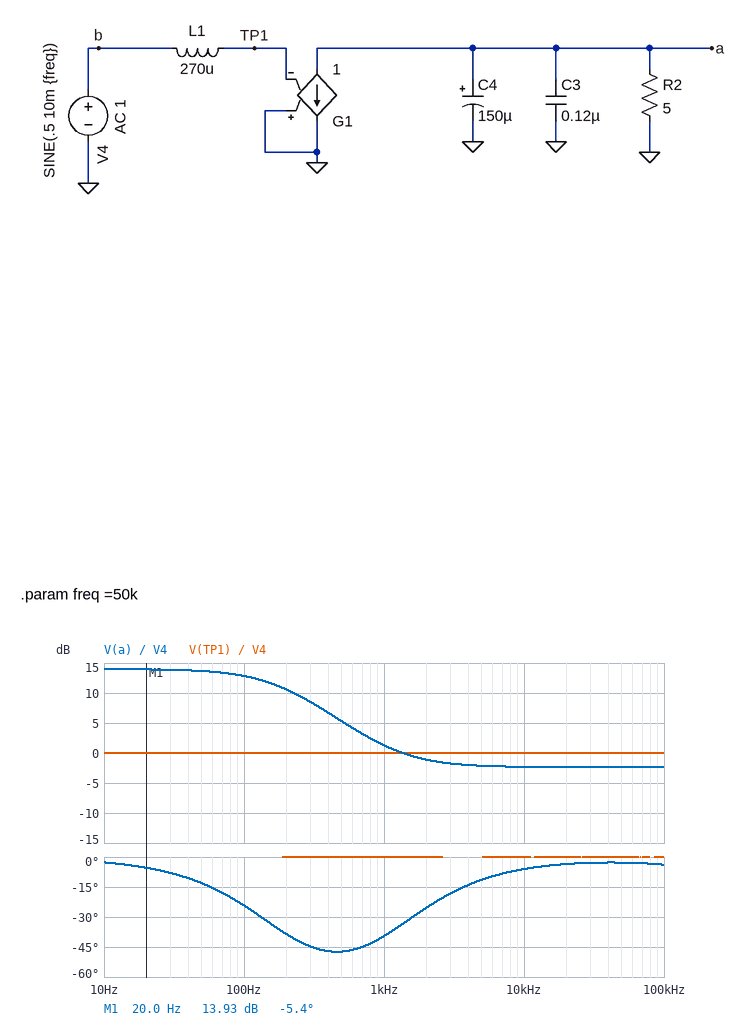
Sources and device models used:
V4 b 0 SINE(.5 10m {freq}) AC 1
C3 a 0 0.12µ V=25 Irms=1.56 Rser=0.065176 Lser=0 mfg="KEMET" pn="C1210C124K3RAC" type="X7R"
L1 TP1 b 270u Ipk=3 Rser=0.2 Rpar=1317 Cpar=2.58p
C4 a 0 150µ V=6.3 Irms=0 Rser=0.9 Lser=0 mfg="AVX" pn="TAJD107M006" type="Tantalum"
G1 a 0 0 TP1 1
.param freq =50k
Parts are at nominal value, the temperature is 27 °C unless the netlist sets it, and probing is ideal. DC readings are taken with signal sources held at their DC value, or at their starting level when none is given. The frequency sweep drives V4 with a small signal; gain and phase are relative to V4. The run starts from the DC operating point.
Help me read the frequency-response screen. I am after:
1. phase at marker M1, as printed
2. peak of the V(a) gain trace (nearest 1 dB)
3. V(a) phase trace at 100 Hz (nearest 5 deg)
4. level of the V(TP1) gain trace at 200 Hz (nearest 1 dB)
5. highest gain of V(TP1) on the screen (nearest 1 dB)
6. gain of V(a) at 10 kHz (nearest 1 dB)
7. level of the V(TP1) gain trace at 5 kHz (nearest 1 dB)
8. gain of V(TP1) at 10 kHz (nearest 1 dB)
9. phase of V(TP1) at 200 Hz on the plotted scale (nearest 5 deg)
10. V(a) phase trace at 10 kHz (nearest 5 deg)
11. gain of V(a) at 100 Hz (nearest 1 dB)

-5.4 deg
14 dB
-25 deg
0 dB
0 dB
-2 dB
0 dB
0 dB
0 deg
-5 deg
13 dB
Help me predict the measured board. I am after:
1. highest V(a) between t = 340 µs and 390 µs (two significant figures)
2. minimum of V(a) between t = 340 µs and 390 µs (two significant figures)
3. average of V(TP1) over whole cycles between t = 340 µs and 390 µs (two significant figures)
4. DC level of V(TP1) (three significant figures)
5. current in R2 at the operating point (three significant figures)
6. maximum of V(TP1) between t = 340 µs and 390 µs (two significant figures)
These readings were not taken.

2.5 V
2.5 V
500 mV
500 mV
500 mA
510 mV
